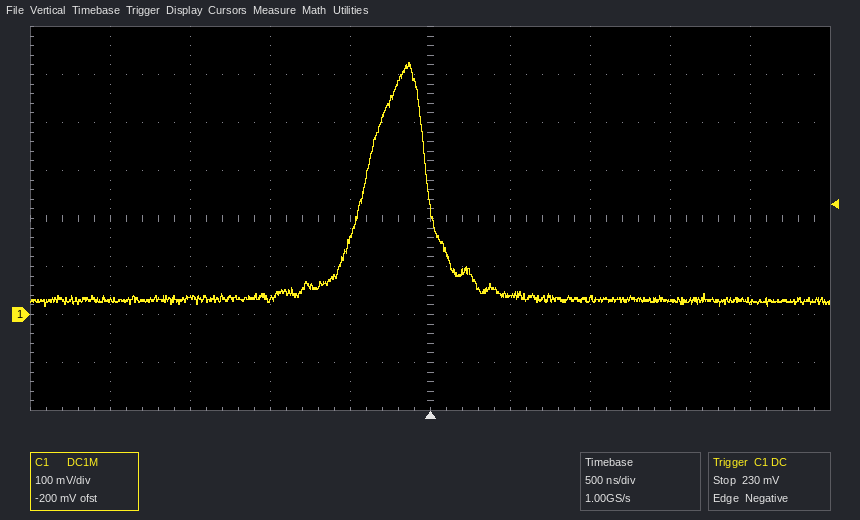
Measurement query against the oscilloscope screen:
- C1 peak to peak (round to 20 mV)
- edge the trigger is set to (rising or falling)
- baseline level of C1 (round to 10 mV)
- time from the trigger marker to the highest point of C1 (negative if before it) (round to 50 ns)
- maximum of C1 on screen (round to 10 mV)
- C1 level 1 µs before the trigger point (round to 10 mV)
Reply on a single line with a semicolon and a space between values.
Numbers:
500 mV; falling; 30 mV; -150 ns; 520 mV; 30 mV
